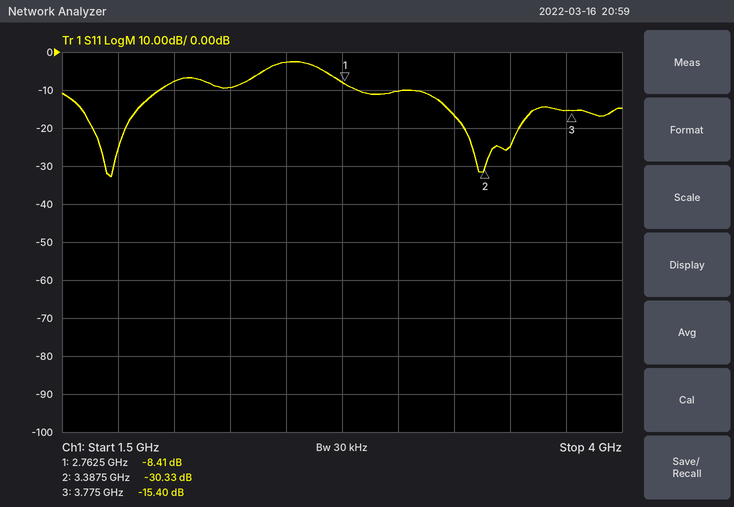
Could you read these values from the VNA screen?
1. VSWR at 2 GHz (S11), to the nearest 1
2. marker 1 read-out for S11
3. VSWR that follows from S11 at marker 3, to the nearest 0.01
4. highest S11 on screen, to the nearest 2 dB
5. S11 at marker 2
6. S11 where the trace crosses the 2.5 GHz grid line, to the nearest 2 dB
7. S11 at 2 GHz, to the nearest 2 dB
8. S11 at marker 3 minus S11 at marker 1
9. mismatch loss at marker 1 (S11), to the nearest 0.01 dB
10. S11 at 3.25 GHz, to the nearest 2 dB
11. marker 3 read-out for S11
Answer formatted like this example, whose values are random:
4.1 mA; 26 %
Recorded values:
2; -8.41 dB; 1.41; -2 dB; -30.33 dB; -2 dB; -8 dB; -6.99 dB; 0.68 dB; -16 dB; -15.40 dB
